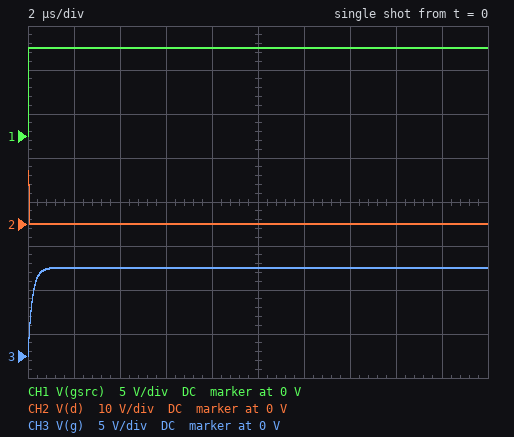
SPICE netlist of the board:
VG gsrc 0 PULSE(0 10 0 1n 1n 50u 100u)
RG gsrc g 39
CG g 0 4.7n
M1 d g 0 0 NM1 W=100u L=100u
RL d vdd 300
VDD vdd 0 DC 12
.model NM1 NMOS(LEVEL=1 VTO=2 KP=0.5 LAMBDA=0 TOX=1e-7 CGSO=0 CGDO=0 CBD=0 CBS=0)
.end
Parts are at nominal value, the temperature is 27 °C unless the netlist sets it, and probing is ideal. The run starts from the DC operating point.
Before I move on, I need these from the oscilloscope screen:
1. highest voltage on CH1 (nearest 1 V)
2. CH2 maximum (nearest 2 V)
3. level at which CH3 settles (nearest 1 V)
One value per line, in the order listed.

10 V
12 V
10 V
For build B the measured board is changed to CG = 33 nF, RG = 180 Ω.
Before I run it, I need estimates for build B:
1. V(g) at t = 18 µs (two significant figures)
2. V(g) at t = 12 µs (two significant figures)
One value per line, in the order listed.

9.5 V
8.7 V
